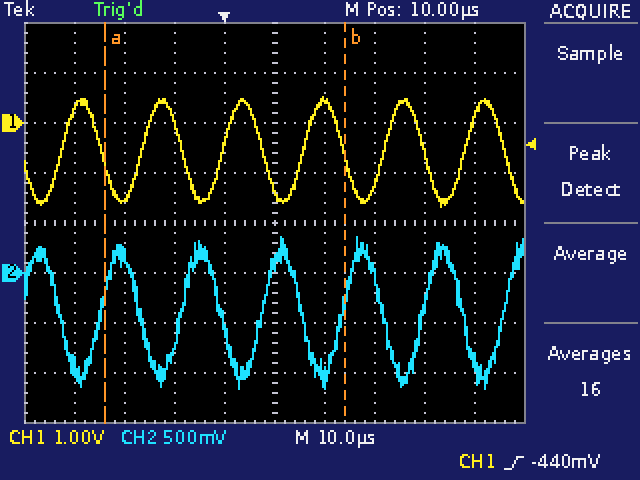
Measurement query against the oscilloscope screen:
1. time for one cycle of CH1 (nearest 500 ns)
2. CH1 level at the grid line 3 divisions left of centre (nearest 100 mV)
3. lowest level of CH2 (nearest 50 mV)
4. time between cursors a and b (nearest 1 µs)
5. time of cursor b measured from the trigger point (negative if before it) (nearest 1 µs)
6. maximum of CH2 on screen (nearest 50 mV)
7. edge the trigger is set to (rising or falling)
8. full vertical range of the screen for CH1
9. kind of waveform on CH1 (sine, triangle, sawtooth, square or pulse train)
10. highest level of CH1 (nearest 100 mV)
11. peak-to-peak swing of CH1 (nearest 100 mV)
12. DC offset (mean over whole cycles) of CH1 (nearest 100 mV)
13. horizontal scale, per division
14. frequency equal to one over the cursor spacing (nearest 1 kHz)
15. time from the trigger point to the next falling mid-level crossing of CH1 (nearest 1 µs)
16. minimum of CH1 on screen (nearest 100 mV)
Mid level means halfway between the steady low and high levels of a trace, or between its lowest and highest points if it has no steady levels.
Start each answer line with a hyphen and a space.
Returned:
- 16.0 µs
- -1.5 V
- -1.15 V
- 48 µs
- +24 µs
- 350 mV
- rising
- 8 V
- sine
- 500 mV
- 2.2 V
- -600 mV
- 10 µs
- 21 kHz
- 8 µs
- -1.7 V
